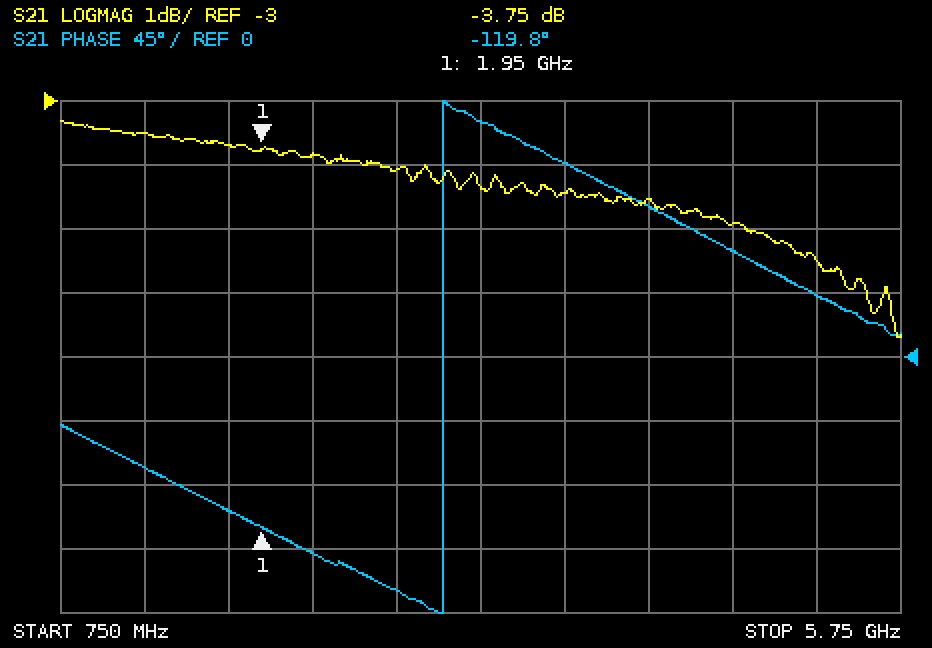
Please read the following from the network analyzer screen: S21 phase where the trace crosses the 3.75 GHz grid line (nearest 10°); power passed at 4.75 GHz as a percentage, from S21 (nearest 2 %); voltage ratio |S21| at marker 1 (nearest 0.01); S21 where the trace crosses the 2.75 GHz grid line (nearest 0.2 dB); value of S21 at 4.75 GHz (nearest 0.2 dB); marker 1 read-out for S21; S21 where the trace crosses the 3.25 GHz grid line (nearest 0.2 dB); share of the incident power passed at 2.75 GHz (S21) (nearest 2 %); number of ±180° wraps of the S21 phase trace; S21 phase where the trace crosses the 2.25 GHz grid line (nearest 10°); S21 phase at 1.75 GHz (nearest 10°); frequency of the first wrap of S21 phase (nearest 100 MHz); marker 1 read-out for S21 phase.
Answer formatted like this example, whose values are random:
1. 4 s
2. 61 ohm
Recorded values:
1. 140°
2. 32 %
3. 0.65
4. -4.0 dB
5. -5.0 dB
6. -3.75 dB
7. -4.4 dB
8. 40 %
9. 1
10. -140°
11. -110°
12. 3.0 GHz
13. -119.8°
